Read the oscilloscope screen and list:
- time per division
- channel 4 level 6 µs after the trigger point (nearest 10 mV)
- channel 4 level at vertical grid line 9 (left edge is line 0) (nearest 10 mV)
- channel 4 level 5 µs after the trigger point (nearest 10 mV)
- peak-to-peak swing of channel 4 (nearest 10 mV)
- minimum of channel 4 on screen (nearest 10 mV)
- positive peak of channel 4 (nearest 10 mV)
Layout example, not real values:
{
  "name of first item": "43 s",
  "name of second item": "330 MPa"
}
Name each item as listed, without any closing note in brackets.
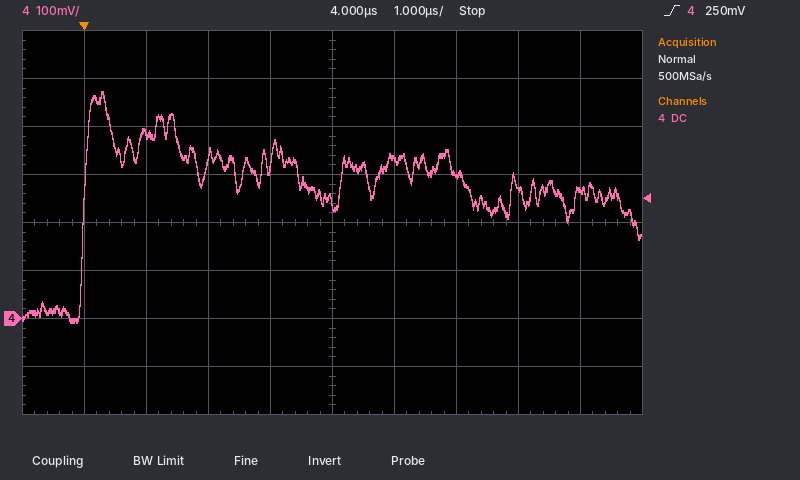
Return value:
{
  "time per division": "1 µs",
  "channel 4 level 6 µs after the trigger point": "300 mV",
  "channel 4 level at vertical grid line 9 (left edge is line 0)": "270 mV",
  "channel 4 level 5 µs after the trigger point": "330 mV",
  "peak-to-peak swing of channel 4": "480 mV",
  "minimum of channel 4 on screen": "-10 mV",
  "positive peak of channel 4": "470 mV"
}
